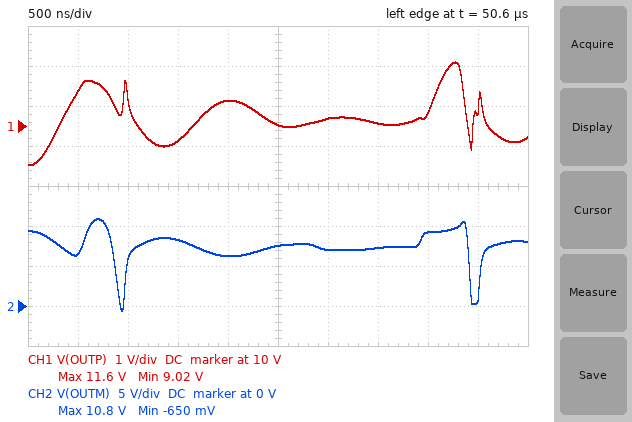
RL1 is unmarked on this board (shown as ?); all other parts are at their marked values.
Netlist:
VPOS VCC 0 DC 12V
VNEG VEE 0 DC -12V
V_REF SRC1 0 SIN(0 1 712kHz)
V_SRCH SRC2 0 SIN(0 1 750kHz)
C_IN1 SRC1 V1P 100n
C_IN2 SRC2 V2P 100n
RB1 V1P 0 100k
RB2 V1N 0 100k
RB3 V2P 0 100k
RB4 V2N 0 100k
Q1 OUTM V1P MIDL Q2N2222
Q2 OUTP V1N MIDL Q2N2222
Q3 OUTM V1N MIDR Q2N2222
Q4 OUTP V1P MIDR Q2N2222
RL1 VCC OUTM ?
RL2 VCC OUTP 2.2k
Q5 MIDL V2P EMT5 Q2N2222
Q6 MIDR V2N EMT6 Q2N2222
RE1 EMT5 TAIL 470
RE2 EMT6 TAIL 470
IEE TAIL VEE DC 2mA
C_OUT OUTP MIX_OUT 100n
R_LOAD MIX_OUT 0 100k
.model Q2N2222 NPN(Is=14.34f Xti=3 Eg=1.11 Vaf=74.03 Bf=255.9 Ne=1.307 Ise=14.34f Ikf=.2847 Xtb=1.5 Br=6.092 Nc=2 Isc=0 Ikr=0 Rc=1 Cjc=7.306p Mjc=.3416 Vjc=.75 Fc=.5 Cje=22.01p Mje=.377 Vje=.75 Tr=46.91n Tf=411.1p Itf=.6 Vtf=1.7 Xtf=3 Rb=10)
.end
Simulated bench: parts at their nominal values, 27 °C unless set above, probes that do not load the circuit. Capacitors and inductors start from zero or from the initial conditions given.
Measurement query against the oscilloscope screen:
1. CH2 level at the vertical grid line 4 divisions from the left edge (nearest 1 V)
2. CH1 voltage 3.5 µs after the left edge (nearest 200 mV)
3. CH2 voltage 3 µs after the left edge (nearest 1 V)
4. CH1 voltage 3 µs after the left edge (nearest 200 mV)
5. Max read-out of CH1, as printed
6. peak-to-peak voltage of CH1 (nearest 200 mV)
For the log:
6 V
10.0 V
7 V
10.2 V
11.6 V
2.6 V
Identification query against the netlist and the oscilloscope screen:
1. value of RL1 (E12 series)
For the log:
3.9 kΩ
